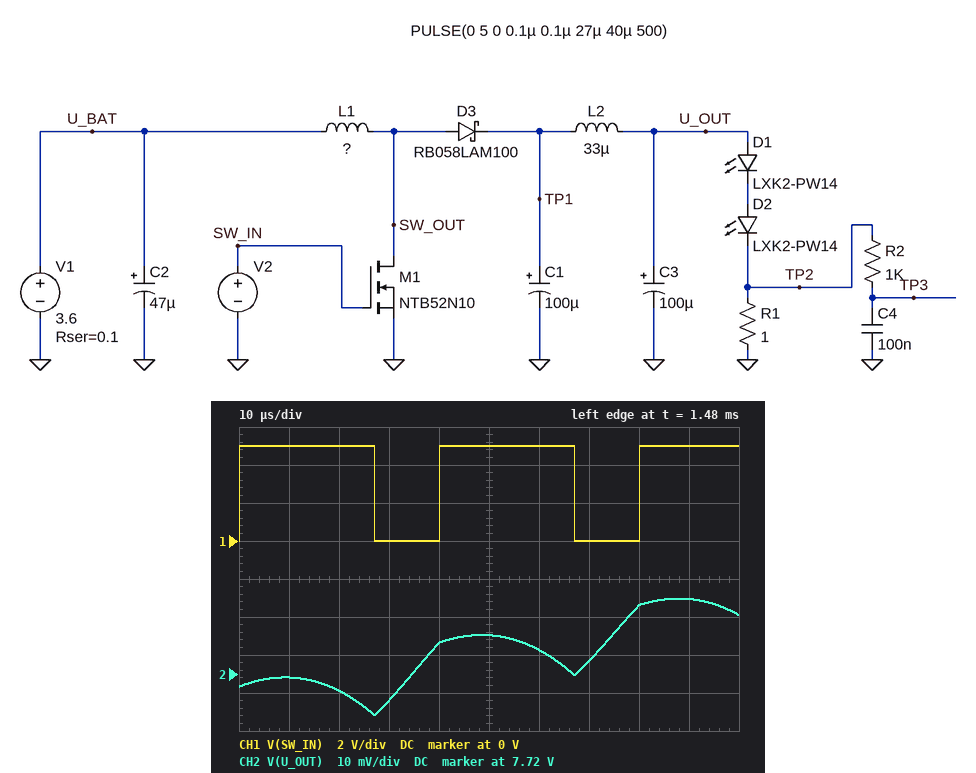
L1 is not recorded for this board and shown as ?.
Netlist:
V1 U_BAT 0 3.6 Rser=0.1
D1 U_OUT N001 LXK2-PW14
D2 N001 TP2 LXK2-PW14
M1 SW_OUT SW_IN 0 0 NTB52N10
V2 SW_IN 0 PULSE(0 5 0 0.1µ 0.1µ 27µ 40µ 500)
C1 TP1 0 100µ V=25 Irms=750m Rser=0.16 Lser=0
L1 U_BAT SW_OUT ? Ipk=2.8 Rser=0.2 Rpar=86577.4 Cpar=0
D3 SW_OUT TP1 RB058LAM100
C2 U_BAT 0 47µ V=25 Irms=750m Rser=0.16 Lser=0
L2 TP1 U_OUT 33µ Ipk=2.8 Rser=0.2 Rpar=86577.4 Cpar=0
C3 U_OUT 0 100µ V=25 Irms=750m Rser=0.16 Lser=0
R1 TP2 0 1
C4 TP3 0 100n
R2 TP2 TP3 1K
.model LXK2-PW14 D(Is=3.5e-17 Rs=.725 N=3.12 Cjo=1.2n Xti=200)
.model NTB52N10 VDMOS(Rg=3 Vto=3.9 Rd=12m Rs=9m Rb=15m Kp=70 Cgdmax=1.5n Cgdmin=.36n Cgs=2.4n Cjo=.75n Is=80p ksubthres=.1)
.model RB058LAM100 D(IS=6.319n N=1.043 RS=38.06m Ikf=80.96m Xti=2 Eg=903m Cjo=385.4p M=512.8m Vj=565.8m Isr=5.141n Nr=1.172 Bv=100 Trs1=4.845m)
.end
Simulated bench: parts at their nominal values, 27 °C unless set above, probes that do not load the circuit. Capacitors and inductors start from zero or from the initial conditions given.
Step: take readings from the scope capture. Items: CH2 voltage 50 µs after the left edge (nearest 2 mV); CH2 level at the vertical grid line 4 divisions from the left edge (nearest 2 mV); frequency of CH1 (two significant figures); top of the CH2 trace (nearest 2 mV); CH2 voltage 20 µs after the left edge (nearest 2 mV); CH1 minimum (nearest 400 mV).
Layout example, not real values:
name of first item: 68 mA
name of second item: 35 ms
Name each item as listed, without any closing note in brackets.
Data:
CH2 voltage 50 µs after the left edge: 7.730 V
CH2 level at the vertical grid line 4 divisions from the left edge: 7.728 V
frequency of CH1: 25 kHz
top of the CH2 trace: 7.740 V
CH2 voltage 20 µs after the left edge: 7.716 V
CH1 minimum: 0 V
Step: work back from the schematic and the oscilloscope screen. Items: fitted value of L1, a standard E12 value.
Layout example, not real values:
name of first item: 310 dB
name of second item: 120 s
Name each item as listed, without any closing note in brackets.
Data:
fitted value of L1, a standard E12 value: 39 µH
